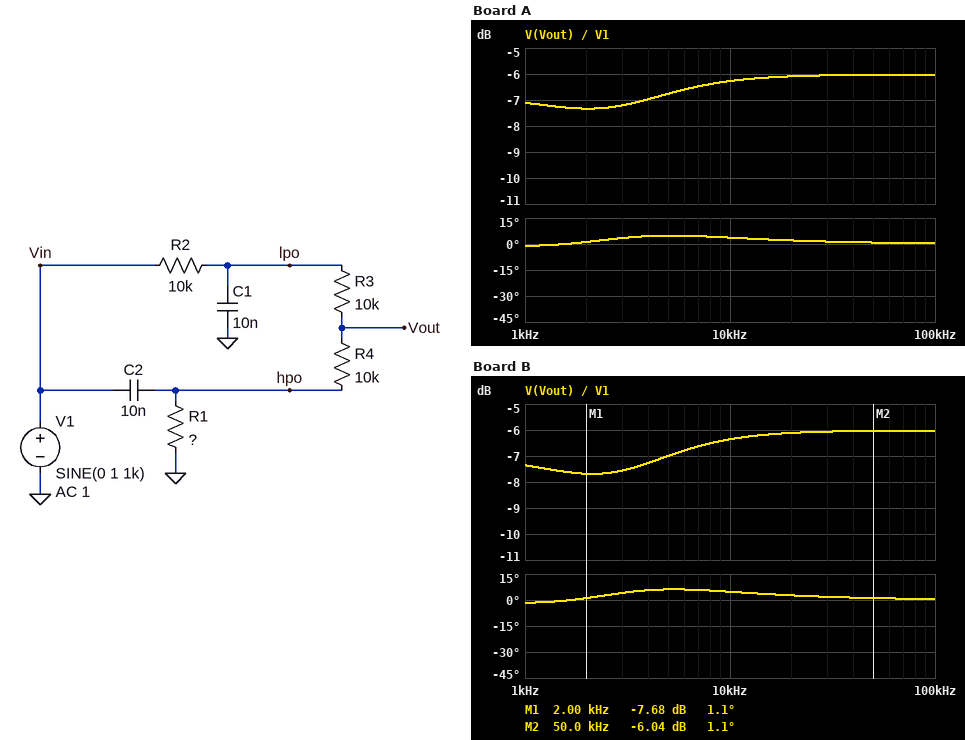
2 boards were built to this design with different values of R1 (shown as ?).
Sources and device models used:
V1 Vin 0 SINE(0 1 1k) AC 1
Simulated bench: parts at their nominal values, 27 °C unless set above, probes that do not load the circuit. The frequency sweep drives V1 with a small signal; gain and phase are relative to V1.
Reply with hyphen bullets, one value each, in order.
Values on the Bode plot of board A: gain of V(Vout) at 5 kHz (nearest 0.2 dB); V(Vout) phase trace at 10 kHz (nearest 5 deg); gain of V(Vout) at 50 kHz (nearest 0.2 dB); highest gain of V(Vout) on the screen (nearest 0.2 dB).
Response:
- -6.8 dB
- 5 deg
- -6.0 dB
- -6.0 dB
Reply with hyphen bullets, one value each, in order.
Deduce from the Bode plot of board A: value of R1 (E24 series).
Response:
- 6.8 kΩ
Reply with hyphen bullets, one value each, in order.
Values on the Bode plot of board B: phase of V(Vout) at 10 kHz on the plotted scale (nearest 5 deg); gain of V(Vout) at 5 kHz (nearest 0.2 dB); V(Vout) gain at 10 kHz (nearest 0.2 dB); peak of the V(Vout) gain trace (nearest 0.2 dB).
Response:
- 5 deg
- -7.0 dB
- -6.4 dB
- -6.0 dB
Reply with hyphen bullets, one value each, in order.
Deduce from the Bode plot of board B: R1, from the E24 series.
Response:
- 6.2 kΩ
